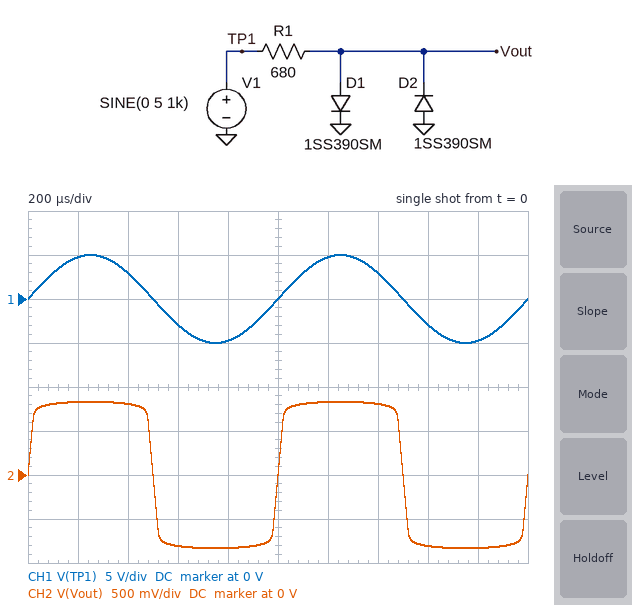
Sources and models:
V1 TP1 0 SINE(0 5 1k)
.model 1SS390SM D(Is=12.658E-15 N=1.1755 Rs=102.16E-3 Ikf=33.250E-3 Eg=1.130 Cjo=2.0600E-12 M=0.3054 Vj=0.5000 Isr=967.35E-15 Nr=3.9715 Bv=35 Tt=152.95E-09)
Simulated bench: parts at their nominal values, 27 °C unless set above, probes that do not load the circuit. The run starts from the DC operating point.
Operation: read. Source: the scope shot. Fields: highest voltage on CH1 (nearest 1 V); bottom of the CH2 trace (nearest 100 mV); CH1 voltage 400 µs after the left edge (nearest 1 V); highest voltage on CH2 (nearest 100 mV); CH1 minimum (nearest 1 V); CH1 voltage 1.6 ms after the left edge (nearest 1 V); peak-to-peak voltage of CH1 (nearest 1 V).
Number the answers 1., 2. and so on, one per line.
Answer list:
1. 5 V
2. -800 mV
3. 3 V
4. 800 mV
5. -5 V
6. -3 V
7. 10 V
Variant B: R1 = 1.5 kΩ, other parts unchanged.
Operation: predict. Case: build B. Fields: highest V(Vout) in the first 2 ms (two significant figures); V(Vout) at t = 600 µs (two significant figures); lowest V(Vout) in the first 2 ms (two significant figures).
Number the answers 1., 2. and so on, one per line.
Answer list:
1. 800 mV
2. -780 mV
3. -800 mV
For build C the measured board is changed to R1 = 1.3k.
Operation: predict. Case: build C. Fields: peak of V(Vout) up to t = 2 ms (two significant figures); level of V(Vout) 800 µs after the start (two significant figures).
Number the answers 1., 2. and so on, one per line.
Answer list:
1. 810 mV
2. -810 mV
